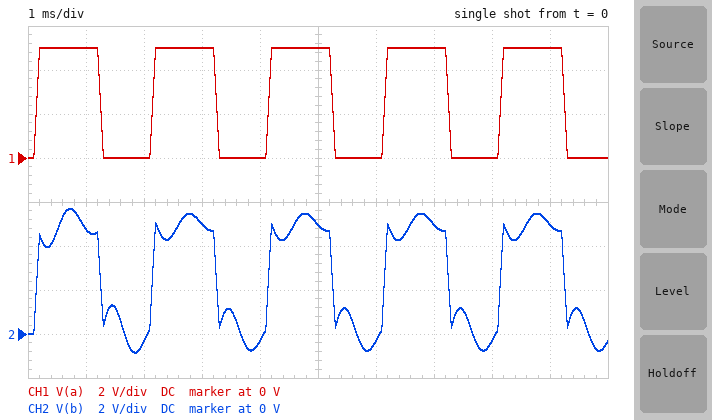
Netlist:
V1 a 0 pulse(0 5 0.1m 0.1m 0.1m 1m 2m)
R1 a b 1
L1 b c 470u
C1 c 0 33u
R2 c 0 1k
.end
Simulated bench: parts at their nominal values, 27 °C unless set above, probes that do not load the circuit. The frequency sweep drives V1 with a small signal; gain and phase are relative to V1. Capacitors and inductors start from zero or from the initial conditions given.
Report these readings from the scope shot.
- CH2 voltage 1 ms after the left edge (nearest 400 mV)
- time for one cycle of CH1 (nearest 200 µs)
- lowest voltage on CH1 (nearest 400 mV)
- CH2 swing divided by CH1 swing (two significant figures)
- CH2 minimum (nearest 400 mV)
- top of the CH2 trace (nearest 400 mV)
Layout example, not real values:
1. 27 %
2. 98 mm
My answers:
1. 4.8 V
2. 2.0 ms
3. 0 V
4. 1.3
5. -800 mV
6. 5.6 V
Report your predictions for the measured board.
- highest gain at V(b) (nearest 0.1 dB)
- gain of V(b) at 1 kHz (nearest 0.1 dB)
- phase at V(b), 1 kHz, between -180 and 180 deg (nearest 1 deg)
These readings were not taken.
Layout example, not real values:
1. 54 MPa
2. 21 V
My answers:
1. 0 dB
2. -1.1 dB
3. -28 deg
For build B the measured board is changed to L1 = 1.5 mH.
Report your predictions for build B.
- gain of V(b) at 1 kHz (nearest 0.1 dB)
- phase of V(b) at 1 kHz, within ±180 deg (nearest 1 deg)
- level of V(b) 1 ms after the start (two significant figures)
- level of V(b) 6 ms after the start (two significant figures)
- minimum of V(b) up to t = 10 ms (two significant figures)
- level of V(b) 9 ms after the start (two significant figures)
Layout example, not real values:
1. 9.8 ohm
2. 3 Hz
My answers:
1. -0.2 dB
2. 12 deg
3. 5.3 V
4. -340 mV
5. -570 mV
6. 5.5 V
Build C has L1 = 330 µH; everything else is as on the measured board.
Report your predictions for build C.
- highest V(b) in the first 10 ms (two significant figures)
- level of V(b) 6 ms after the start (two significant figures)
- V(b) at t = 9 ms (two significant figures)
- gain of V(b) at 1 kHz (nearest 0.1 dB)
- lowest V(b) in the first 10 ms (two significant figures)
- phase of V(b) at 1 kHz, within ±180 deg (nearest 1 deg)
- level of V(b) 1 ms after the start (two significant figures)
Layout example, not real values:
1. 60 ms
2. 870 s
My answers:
1. 5.9 V
2. 460 mV
3. 4.5 V
4. -0.6 dB
5. -870 mV
6. -20 deg
7. 4.6 V
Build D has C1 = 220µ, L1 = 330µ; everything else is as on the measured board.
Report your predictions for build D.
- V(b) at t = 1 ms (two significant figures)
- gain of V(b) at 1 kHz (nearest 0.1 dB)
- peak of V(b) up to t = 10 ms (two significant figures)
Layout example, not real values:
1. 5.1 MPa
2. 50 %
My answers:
1. 4.7 V
2. -1.9 dB
3. 5.5 V
